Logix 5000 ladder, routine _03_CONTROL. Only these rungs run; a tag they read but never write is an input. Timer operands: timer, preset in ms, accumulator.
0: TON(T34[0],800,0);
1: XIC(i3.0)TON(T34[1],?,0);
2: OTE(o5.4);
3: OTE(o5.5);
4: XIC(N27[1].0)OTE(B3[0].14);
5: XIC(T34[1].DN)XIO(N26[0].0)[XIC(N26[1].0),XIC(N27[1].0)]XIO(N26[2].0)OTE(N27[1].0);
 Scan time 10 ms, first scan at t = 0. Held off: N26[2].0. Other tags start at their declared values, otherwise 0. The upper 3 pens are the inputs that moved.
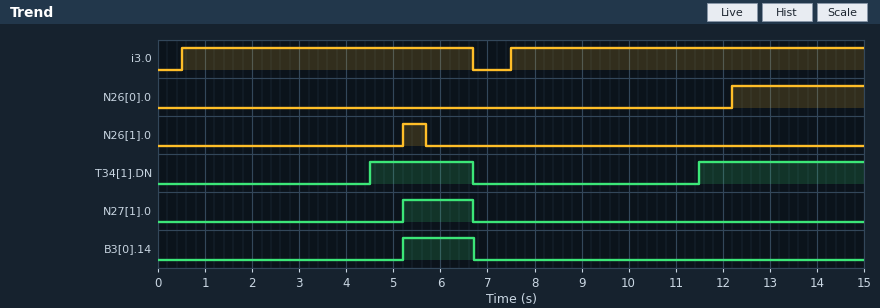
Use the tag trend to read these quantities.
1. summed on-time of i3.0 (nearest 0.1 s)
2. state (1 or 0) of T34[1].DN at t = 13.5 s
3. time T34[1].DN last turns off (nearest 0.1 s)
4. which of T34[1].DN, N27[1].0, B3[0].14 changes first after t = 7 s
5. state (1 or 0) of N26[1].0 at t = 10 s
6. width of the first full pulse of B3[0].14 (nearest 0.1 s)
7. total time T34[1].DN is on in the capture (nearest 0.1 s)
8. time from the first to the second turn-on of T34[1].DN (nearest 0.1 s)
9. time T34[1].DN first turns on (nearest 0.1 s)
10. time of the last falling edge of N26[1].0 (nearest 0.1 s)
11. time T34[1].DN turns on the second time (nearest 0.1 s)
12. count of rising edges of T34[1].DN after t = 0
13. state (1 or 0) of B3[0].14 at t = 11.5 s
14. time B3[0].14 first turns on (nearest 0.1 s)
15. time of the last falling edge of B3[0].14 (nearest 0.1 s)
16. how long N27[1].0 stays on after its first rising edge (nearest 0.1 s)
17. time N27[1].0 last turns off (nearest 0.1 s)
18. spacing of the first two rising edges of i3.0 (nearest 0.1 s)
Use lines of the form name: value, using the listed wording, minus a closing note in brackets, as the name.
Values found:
summed on-time of i3.0: 13.7 s
state (1 or 0) of T34[1].DN at t = 13.5 s: 1
time T34[1].DN last turns off: 6.7 s
which of T34[1].DN, N27[1].0, B3[0].14 changes first after t = 7 s: T34[1].DN
state (1 or 0) of N26[1].0 at t = 10 s: 0
width of the first full pulse of B3[0].14: 1.5 s
total time T34[1].DN is on in the capture: 5.7 s
time from the first to the second turn-on of T34[1].DN: 7.0 s
time T34[1].DN first turns on: 4.5 s
time of the last falling edge of N26[1].0: 5.7 s
time T34[1].DN turns on the second time: 11.5 s
count of rising edges of T34[1].DN after t = 0: 2
state (1 or 0) of B3[0].14 at t = 11.5 s: 0
time B3[0].14 first turns on: 5.2 s
time of the last falling edge of B3[0].14: 6.7 s
how long N27[1].0 stays on after its first rising edge: 1.5 s
time N27[1].0 last turns off: 6.7 s
spacing of the first two rising edges of i3.0: 7.0 s
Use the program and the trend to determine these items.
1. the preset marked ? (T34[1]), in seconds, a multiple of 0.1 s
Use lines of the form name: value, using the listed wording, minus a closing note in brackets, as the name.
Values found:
the preset marked ? (T34[1]), in seconds, a multiple of 0.1 s: 4.0 s
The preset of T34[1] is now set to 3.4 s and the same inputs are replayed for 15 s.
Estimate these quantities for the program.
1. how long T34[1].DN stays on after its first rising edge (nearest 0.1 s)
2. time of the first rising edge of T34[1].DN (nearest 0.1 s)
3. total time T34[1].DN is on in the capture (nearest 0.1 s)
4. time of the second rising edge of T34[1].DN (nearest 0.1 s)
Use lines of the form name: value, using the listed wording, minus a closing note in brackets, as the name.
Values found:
how long T34[1].DN stays on after its first rising edge: 2.8 s
time of the first rising edge of T34[1].DN: 3.9 s
total time T34[1].DN is on in the capture: 6.9 s
time of the second rising edge of T34[1].DN: 10.9 s
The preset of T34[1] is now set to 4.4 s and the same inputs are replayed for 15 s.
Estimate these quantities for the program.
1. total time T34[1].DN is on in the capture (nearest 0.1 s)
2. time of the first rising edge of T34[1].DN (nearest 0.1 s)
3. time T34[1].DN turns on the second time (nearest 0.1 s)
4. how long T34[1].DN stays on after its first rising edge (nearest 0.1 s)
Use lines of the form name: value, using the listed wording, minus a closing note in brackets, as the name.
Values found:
total time T34[1].DN is on in the capture: 4.9 s
time of the first rising edge of T34[1].DN: 4.9 s
time T34[1].DN turns on the second time: 11.9 s
how long T34[1].DN stays on after its first rising edge: 1.8 s
